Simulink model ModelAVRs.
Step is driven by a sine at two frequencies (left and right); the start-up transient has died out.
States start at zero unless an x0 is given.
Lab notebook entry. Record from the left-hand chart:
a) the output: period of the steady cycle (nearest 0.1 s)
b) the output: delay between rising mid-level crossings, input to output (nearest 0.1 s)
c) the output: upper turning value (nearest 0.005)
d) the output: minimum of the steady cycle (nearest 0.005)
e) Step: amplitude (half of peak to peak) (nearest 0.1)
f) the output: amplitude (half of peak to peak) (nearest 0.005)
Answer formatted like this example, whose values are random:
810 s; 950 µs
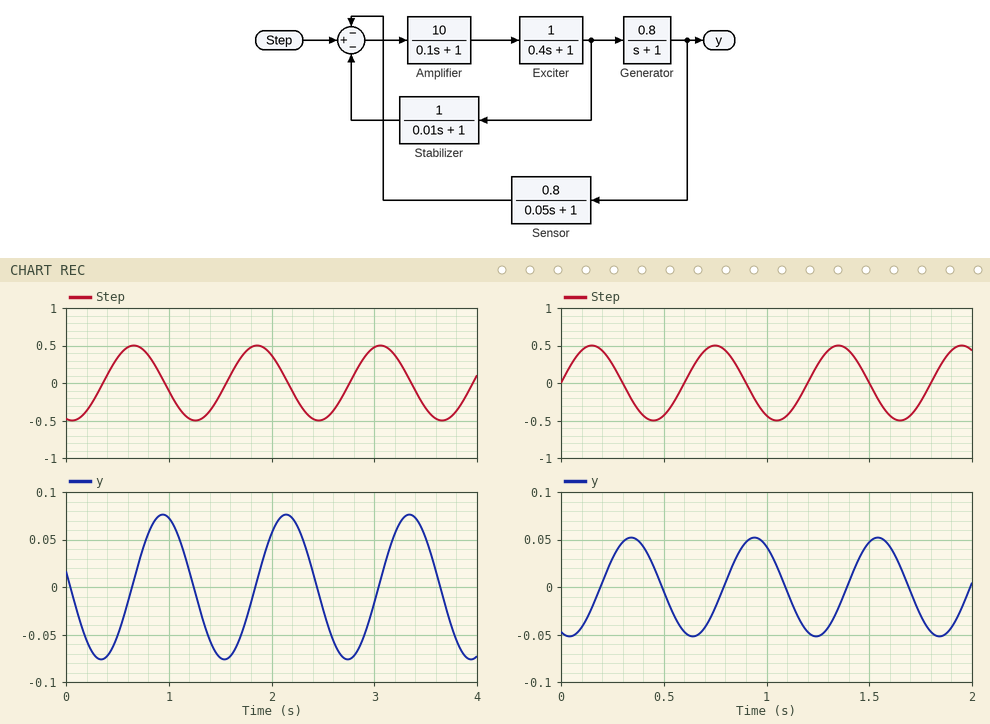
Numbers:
1.2 s; 0.3 s; 0.075; -0.075; 0.5; 0.075
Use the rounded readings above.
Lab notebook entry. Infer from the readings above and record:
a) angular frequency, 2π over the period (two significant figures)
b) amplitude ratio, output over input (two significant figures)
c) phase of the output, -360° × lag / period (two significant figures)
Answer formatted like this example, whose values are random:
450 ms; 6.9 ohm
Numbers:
5.2 rad/s; 0.15; -90°
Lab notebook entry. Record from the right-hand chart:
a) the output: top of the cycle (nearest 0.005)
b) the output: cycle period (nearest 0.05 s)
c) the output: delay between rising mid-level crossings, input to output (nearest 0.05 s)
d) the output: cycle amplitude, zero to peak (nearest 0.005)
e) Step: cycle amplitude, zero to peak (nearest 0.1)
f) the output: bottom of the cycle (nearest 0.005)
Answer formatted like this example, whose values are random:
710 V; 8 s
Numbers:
0.050; 0.60 s; 0.20 s; 0.050; 0.5; -0.050
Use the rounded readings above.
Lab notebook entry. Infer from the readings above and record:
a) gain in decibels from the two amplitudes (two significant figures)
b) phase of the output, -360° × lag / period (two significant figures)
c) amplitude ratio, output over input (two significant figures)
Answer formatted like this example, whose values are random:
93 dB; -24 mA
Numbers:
-20 dB; -120°; 0.10
